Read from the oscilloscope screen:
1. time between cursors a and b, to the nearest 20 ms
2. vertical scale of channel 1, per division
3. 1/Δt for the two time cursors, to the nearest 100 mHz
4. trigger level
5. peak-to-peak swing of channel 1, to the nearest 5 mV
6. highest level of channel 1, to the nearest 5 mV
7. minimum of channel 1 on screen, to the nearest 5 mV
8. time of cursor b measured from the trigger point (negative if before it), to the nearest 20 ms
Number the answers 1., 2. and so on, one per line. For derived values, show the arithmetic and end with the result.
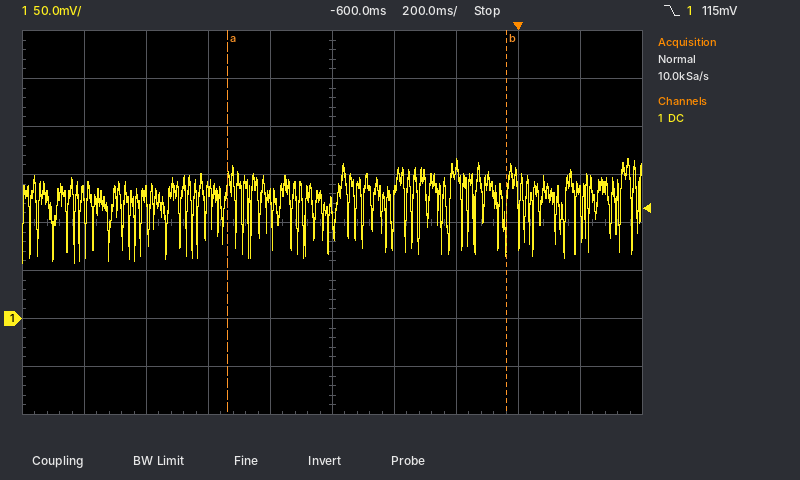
1. 900 ms
2. 50 mV
3. 1 / 900 ms ≈ 1.1 Hz
4. 115 mV
5. 165 mV − (55 mV) = 110 mV
6. 165 mV
7. 55 mV
8. -40 ms
